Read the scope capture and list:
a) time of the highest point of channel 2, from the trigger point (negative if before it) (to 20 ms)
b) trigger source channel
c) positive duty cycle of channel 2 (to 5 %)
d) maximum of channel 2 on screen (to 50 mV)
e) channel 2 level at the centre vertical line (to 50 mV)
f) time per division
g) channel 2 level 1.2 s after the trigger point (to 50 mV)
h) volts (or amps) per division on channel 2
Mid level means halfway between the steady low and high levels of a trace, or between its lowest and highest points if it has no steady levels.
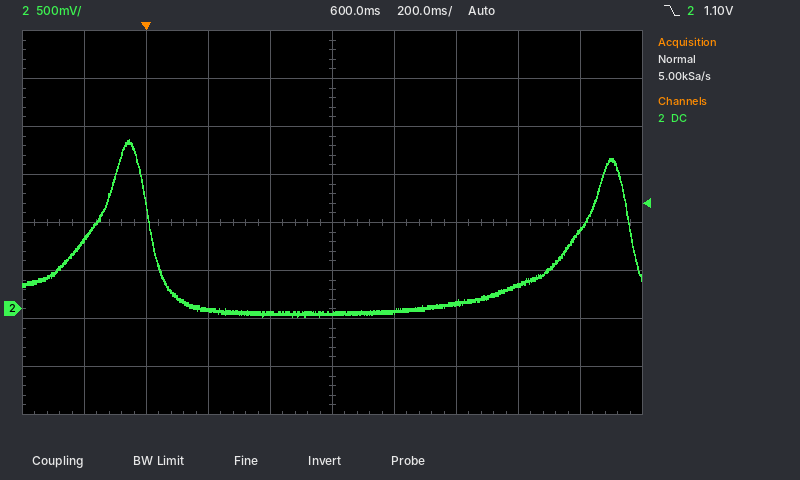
-60 ms
channel 2
10 %
1.75 V
-50 mV
200 ms
250 mV
500 mV
